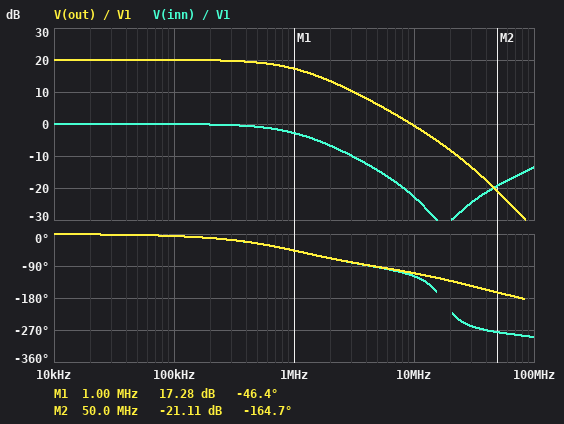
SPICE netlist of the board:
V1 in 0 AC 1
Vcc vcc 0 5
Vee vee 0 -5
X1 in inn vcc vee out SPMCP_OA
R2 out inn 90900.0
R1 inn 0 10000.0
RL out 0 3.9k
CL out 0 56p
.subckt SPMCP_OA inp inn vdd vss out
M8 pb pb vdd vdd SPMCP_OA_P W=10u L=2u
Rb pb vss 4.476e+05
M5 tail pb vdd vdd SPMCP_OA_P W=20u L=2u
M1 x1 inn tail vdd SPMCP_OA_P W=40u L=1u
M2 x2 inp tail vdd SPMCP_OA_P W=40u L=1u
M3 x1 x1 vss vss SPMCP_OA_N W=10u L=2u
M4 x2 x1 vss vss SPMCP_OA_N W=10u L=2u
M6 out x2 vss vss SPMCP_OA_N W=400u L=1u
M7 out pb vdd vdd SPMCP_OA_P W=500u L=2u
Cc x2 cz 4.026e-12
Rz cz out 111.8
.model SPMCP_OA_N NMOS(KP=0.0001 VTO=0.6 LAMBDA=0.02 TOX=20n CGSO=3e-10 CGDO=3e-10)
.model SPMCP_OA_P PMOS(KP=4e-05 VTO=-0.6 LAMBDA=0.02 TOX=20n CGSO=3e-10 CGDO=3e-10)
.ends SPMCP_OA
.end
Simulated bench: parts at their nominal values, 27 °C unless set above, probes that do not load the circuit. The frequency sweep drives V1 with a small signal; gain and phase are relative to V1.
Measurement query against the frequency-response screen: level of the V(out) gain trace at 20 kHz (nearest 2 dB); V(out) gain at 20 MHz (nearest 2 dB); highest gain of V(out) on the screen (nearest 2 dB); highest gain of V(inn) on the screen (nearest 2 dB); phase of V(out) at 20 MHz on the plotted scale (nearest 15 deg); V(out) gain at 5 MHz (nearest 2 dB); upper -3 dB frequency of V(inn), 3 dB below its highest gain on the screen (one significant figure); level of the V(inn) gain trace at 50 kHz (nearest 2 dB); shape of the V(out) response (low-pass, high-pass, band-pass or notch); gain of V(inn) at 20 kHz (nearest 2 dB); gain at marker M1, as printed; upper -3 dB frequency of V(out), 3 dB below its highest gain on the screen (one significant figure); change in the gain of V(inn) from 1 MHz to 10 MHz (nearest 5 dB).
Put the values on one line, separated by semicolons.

20 dB; -8 dB; 20 dB; 0 dB; -135 deg; 6 dB; 1 MHz; 0 dB; low-pass; 0 dB; 17.28 dB; 1 MHz; -20 dB
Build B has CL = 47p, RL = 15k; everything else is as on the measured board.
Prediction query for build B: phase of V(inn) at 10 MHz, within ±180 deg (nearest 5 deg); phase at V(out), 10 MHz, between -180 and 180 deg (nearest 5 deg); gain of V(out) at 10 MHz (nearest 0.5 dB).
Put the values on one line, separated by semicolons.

-115 deg; -105 deg; 0 dB
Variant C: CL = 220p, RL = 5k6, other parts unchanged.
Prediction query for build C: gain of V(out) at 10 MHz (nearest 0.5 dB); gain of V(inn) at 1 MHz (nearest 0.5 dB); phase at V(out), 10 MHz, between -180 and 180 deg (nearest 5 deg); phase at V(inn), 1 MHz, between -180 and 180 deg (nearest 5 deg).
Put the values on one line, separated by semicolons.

-5.0 dB; -2.5 dB; -150 deg; -50 deg
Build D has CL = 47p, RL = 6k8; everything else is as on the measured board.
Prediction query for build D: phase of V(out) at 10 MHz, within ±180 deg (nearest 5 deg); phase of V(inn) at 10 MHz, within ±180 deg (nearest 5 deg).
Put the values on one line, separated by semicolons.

-105 deg; -115 deg
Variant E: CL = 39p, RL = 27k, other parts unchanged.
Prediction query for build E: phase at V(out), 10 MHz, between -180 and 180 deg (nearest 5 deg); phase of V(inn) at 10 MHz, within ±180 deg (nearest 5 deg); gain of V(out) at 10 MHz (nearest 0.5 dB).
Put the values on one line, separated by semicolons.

-105 deg; -110 deg; 0 dB
